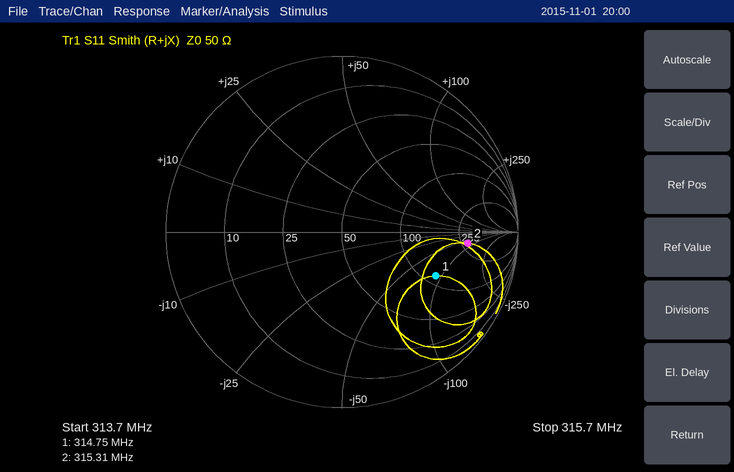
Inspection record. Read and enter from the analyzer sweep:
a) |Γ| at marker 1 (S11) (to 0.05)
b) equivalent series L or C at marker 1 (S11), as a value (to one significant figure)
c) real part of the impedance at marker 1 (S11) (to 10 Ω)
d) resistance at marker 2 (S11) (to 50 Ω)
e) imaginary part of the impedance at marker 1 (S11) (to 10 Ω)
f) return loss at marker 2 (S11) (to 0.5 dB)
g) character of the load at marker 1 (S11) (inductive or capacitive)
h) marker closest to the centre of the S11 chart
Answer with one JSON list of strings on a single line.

["0.60", "6 pF", "120 Ω", "300 Ω", "-90 Ω", "3.0 dB", "capacitive", "marker 1"]
